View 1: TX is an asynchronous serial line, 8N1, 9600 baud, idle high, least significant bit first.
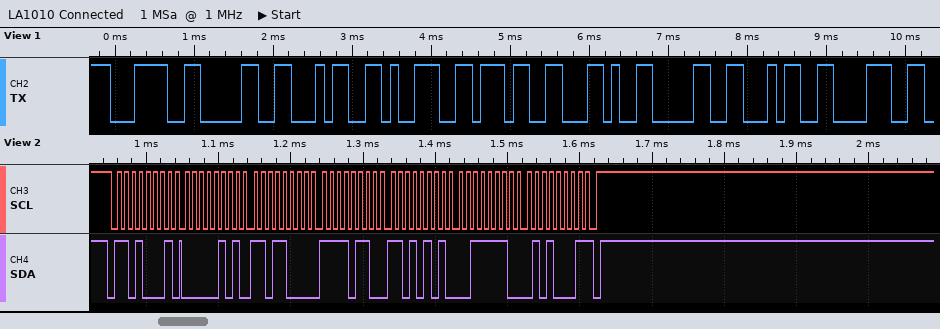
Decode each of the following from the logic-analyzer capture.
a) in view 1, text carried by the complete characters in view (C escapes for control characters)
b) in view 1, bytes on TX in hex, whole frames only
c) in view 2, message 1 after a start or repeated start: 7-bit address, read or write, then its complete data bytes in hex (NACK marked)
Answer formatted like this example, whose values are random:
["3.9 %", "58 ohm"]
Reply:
["\"<0497,048\"", "3C 30 34 39 37 2C 30 34 38", "0x68 read: 05 D8 F6 D5 3E 51 NACK"]
